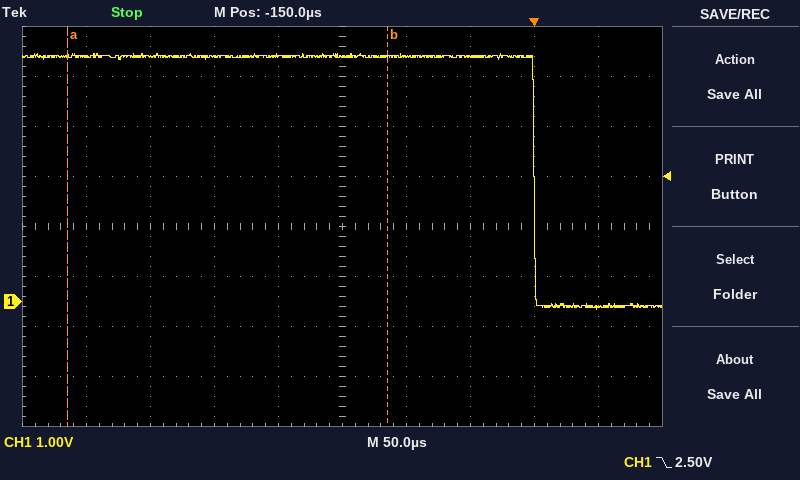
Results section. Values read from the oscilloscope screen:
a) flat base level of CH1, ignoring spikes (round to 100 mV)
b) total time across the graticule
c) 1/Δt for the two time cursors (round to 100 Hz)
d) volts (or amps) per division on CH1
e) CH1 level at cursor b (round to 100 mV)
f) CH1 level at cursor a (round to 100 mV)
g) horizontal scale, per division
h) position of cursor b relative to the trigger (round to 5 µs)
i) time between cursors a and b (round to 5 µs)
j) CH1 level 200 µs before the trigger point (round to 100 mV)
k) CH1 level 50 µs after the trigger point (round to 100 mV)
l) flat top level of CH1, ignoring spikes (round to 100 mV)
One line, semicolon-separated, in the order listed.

-100 mV; 500 µs; 4.0 kHz; 1 V; 4.9 V; 4.9 V; 50 µs; -115 µs; 250 µs; 4.9 V; -100 mV; 4.9 V
